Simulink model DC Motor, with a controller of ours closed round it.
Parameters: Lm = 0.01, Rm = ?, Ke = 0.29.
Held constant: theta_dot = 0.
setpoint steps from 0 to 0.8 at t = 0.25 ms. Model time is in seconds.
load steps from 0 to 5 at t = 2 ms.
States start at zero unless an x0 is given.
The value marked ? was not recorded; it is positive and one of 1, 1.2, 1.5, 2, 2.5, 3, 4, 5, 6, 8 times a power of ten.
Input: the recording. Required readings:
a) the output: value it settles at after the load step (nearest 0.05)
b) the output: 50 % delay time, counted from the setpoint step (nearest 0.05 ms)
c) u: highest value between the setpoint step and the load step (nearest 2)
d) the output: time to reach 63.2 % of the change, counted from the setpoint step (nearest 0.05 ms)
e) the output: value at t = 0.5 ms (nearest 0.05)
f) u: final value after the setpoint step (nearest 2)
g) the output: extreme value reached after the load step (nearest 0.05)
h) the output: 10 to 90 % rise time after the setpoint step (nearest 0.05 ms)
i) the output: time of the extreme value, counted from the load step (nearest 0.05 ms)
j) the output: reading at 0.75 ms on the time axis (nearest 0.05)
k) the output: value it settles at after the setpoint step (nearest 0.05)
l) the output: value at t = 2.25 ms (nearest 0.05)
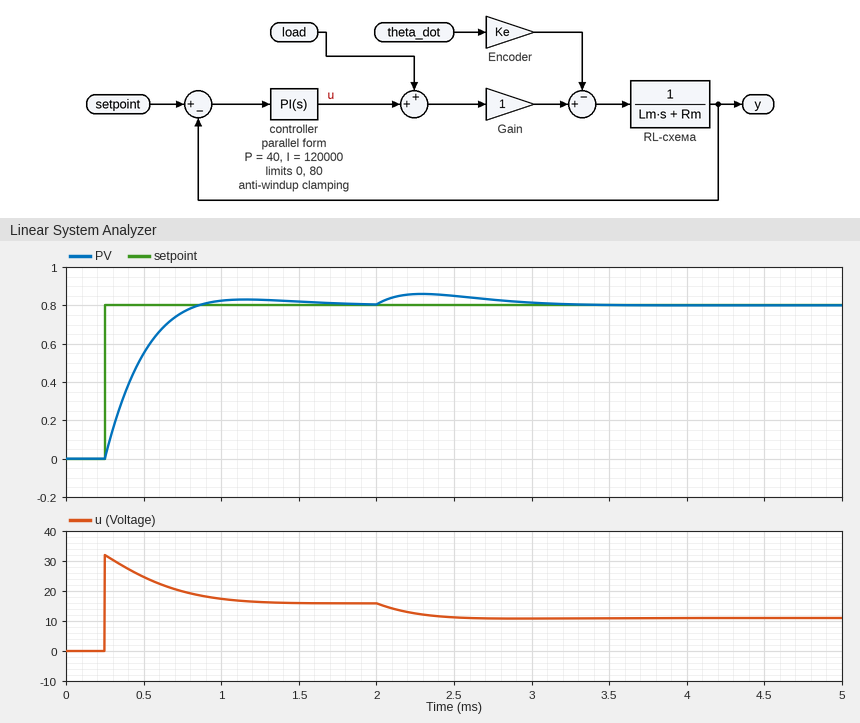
0.80
0.15 ms
32
0.20 ms
0.55
16
0.85
0.40 ms
0.30 ms
0.75
0.80
0.85
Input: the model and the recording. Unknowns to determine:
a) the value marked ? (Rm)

20
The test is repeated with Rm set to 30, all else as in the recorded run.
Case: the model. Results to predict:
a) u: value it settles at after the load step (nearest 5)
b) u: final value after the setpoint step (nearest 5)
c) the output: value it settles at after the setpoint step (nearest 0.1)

20
25
0.8
